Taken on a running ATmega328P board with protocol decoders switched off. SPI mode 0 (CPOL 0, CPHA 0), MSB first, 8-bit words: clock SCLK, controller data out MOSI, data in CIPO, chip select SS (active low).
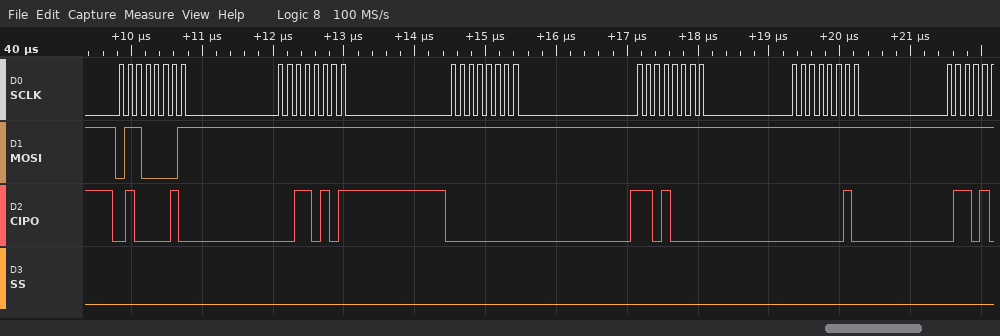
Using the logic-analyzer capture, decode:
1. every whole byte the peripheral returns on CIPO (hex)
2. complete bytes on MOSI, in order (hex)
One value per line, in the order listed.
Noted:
42 35 00 D0 02
61 FF FF FF FF
